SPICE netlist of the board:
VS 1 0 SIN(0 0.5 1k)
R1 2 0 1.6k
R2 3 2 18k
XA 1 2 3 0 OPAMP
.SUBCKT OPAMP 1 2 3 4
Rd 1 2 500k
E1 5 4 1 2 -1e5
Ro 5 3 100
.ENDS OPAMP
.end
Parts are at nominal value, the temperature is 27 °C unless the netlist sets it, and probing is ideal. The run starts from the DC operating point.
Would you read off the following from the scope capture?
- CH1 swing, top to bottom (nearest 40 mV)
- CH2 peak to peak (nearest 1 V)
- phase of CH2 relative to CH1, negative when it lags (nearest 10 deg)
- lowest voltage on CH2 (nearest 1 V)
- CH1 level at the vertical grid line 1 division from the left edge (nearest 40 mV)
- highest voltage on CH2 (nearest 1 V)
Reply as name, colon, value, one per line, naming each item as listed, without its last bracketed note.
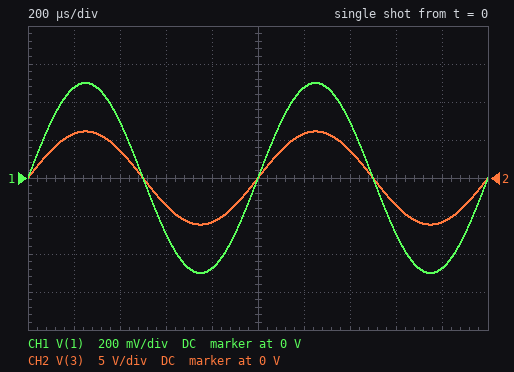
CH1 swing, top to bottom: 1.00 V
CH2 peak to peak: 12 V
phase of CH2 relative to CH1, negative when it lags: 0 deg
lowest voltage on CH2: -6 V
CH1 level at the vertical grid line 1 division from the left edge: 480 mV
highest voltage on CH2: 6 V
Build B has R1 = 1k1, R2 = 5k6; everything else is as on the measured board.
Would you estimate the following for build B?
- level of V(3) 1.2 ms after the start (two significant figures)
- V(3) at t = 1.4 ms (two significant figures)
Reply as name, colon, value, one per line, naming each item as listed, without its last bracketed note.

level of V(3) 1.2 ms after the start: 2.9 V
V(3) at t = 1.4 ms: 1.8 V
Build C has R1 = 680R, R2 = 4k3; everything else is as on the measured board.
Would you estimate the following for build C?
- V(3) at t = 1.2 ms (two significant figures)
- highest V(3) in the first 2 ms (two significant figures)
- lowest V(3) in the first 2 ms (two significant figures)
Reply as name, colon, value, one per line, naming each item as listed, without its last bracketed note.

V(3) at t = 1.2 ms: 3.5 V
highest V(3) in the first 2 ms: 3.7 V
lowest V(3) in the first 2 ms: -3.7 V
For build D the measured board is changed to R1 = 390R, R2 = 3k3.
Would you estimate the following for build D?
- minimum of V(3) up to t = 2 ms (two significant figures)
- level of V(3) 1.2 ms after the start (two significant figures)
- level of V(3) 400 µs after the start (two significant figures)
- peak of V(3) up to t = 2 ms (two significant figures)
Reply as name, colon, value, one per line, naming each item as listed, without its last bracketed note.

minimum of V(3) up to t = 2 ms: -4.7 V
level of V(3) 1.2 ms after the start: 4.5 V
level of V(3) 400 µs after the start: 2.8 V
peak of V(3) up to t = 2 ms: 4.7 V
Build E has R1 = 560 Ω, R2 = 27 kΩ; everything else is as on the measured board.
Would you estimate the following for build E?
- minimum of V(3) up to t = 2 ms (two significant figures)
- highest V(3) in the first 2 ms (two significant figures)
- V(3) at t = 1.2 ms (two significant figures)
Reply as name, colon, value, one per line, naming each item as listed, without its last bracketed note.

minimum of V(3) up to t = 2 ms: -25 V
highest V(3) in the first 2 ms: 25 V
V(3) at t = 1.2 ms: 23 V
